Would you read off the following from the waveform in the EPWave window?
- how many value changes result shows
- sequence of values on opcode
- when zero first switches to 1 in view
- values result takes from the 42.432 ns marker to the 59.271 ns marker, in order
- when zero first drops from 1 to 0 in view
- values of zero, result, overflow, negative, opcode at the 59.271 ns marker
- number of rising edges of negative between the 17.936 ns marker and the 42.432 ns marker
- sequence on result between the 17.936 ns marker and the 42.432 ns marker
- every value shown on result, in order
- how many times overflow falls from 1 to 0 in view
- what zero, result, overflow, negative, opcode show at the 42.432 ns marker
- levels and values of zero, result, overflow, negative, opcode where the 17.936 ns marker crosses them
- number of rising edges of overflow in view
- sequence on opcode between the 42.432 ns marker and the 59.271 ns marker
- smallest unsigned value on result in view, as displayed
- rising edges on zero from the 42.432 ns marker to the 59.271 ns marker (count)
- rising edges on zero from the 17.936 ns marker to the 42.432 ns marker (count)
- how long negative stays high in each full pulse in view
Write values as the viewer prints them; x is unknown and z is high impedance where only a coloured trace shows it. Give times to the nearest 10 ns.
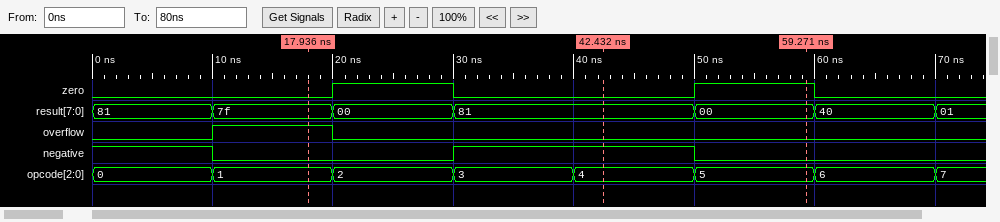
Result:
6
0, 1, 2, 3, 4, 5, 6, 7
20 ns
81, 00
30 ns
zero=1, result=00, overflow=0, negative=0, opcode=5
1
7f, 00, 81
81, 7f, 00, 81, 00, 40, 01
1
zero=0, result=81, overflow=0, negative=1, opcode=4
zero=0, result=7f, overflow=1, negative=0, opcode=1
1
4, 5
00
1
1
20 ns
